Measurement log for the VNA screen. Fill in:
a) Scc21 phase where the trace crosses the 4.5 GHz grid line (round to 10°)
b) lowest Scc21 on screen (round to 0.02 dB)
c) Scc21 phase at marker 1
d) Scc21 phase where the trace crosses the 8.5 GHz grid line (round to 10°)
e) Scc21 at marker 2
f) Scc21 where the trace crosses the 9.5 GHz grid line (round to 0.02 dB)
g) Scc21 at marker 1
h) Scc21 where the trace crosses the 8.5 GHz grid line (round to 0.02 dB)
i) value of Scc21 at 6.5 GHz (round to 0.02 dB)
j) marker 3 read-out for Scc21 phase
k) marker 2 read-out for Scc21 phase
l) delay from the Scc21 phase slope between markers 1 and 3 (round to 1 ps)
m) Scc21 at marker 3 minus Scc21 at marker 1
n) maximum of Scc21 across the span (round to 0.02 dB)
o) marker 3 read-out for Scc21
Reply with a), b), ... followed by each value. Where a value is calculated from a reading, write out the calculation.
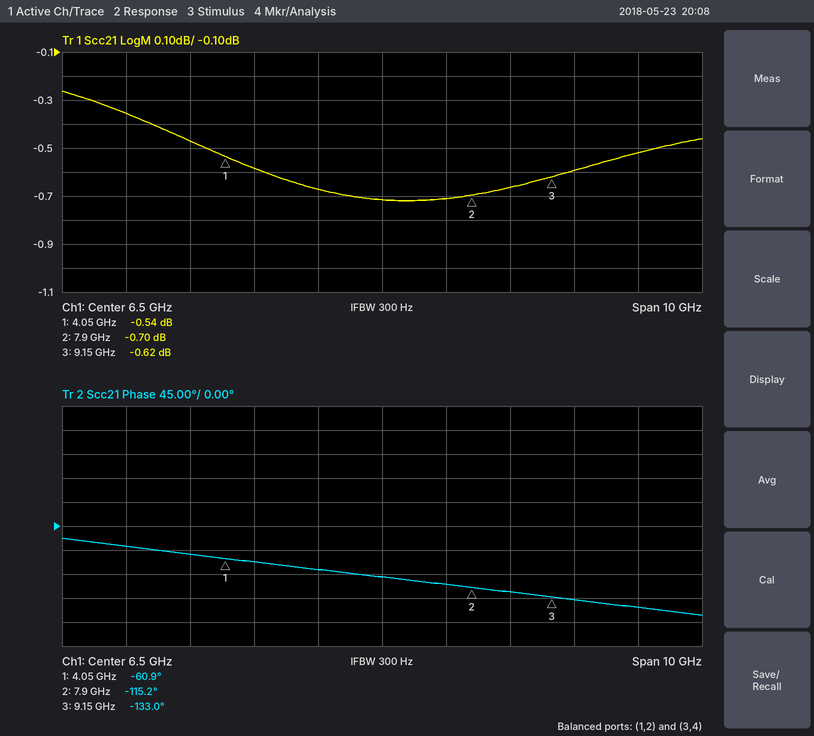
a) -70°
b) -0.72 dB
c) -60.9°
d) -120°
e) -0.70 dB
f) -0.60 dB
g) -0.54 dB
h) -0.66 dB
i) -0.72 dB
j) -133.0°
k) -115.2°
l) −(-133° − (-60.9°))/(360° × 5.1 GHz) ≈ 39 ps
m) -0.62 − (-0.54) = -0.08 dB
n) -0.26 dB
o) -0.62 dB
